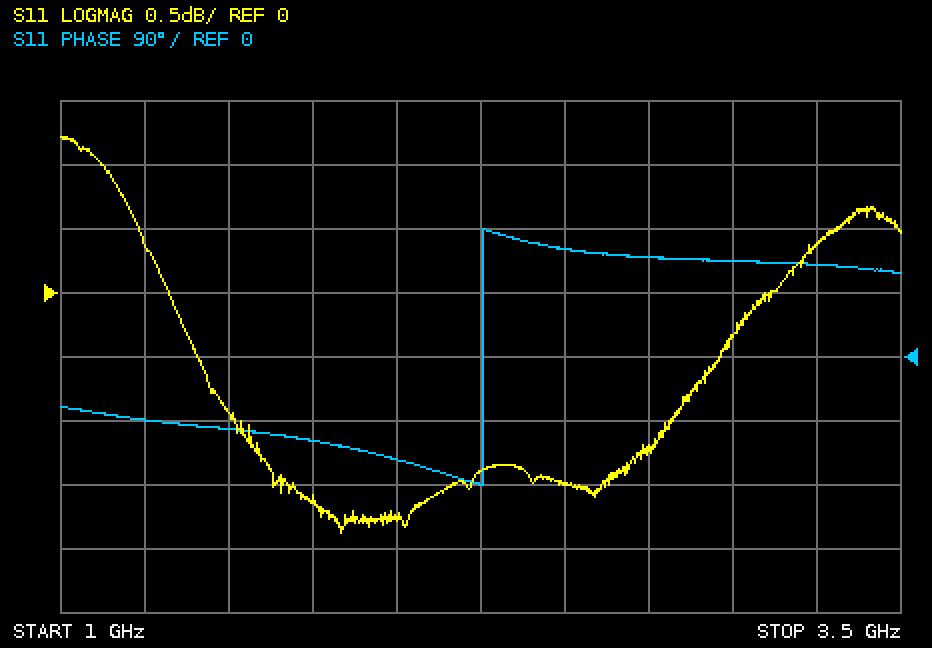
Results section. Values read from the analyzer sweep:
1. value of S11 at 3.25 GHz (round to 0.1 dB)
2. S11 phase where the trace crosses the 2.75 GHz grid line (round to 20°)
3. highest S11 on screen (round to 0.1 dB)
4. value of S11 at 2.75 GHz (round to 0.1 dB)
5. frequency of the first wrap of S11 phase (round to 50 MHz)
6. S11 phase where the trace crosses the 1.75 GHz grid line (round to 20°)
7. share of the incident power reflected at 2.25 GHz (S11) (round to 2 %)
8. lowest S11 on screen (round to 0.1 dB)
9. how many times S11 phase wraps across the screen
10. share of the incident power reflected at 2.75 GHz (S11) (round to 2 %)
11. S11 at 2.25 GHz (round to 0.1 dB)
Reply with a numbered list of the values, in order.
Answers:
1. 0.4 dB
2. 140°
3. 1.2 dB
4. -1.2 dB
5. 2.25 GHz
6. -120°
7. 72 %
8. -1.9 dB
9. 1
10. 76 %
11. -1.4 dB
